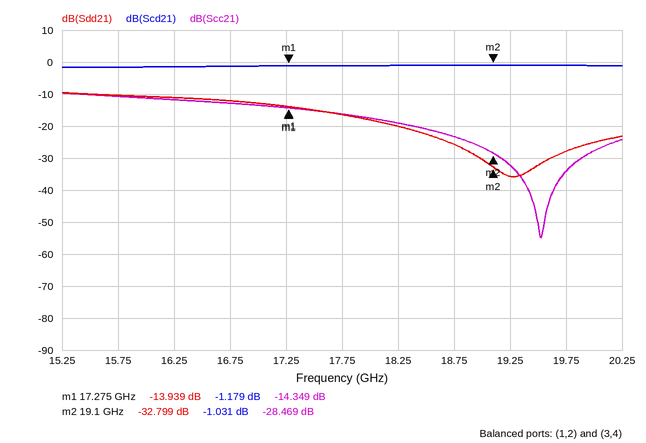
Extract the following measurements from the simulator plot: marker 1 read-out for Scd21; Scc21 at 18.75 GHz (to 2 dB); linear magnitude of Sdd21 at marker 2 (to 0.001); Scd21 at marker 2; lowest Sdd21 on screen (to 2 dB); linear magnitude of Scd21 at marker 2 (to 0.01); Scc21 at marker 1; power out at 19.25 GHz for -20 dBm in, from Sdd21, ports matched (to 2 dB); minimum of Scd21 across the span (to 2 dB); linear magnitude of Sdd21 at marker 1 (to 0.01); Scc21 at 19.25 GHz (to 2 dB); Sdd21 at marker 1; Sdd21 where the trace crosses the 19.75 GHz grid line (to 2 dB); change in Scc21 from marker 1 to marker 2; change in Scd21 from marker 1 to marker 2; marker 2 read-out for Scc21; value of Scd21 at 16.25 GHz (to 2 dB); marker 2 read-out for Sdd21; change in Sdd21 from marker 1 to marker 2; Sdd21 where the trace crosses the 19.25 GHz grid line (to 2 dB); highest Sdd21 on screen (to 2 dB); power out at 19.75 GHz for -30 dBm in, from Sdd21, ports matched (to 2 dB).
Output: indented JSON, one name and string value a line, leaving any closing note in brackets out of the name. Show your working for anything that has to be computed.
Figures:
{
  "marker 1 read-out for Scd21": "-1.179 dB",
  "Scc21 at 18.75 GHz": "-24 dB",
  "linear magnitude of Sdd21 at marker 2": "10^(-32.799/20) ≈ 0.023",
  "Scd21 at marker 2": "-1.031 dB",
  "lowest Sdd21 on screen": "-36 dB",
  "linear magnitude of Scd21 at marker 2": "10^(-1.031/20) ≈ 0.89",
  "Scc21 at marker 1": "-14.349 dB",
  "power out at 19.25 GHz for -20 dBm in, from Sdd21, ports matched": "-20 dBm + (-36 dB) = -56 dBm",
  "minimum of Scd21 across the span": "-2 dB",
  "linear magnitude of Sdd21 at marker 1": "10^(-13.939/20) ≈ 0.20",
  "Scc21 at 19.25 GHz": "-32 dB",
  "Sdd21 at marker 1": "-13.939 dB",
  "Sdd21 where the trace crosses the 19.75 GHz grid line": "-28 dB",
  "change in Scc21 from marker 1 to marker 2": "-28.469 − (-14.349) = -14.120 dB",
  "change in Scd21 from marker 1 to marker 2": "-1.031 − (-1.179) = 0.148 dB",
  "marker 2 read-out for Scc21": "-28.469 dB",
  "value of Scd21 at 16.25 GHz": "-2 dB",
  "marker 2 read-out for Sdd21": "-32.799 dB",
  "change in Sdd21 from marker 1 to marker 2": "-32.799 − (-13.939) = -18.860 dB",
  "Sdd21 where the trace crosses the 19.25 GHz grid line": "-36 dB",
  "highest Sdd21 on screen": "-10 dB",
  "power out at 19.75 GHz for -30 dBm in, from Sdd21, ports matched": "-30 dBm + (-28 dB) = -58 dBm"
}
